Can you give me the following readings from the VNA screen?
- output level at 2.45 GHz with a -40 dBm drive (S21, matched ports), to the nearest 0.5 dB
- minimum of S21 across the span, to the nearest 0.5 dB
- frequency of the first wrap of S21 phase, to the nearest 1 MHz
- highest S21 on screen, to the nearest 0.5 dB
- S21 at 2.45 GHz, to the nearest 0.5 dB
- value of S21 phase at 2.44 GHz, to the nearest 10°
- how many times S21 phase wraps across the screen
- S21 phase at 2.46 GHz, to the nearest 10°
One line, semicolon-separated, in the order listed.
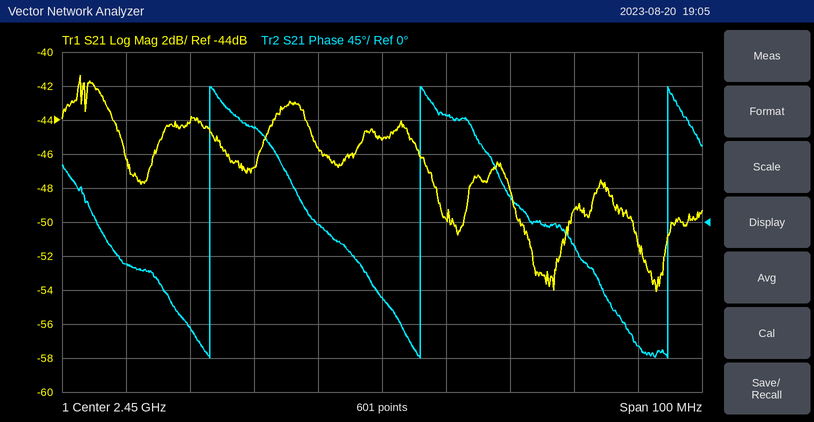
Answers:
-85.0 dBm; -54.0 dB; 2.423 GHz; -41.5 dB; -45.0 dB; 0°; 3; 140°
